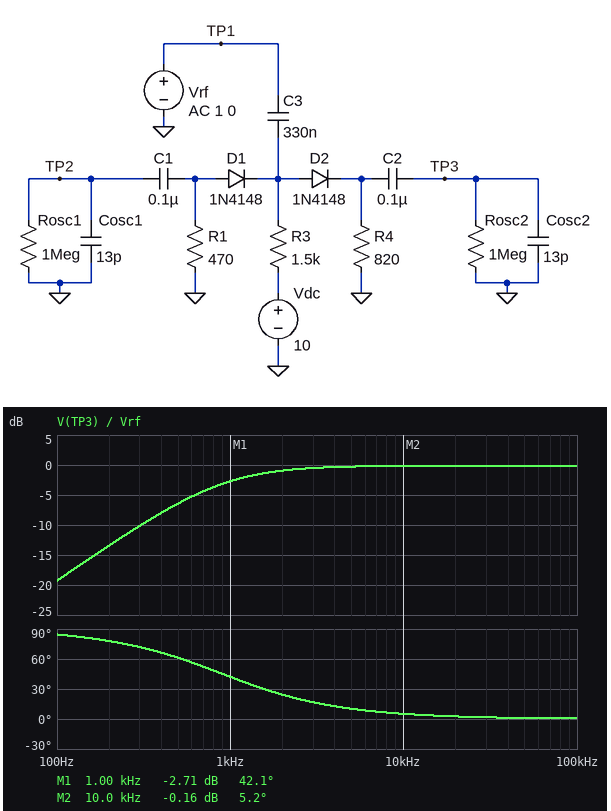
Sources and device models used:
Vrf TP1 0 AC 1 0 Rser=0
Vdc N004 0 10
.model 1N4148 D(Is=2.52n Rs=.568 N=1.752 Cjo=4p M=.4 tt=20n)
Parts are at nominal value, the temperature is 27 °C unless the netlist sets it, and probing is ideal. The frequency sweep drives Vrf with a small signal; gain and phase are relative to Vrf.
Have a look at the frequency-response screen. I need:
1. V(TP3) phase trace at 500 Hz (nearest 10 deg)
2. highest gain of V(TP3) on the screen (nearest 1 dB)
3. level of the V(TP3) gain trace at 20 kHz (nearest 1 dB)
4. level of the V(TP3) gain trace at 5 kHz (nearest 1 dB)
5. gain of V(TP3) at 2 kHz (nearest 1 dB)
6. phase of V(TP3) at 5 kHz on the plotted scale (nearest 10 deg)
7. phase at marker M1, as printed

60 deg
0 dB
0 dB
0 dB
-1 dB
10 deg
42.1 deg
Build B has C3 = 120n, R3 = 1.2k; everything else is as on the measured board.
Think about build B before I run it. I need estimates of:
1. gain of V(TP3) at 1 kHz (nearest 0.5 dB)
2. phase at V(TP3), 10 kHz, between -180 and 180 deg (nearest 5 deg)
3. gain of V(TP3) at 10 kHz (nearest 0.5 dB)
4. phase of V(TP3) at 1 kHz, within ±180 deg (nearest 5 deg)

-9.5 dB
15 deg
-0.5 dB
70 deg
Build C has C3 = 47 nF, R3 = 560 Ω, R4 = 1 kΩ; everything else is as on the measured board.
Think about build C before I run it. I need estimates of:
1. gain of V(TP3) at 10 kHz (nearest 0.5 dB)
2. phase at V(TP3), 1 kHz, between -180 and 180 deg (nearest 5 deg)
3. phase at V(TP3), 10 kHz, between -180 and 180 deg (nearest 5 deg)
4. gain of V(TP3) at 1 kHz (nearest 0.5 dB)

-3.0 dB
85 deg
45 deg
-19.5 dB
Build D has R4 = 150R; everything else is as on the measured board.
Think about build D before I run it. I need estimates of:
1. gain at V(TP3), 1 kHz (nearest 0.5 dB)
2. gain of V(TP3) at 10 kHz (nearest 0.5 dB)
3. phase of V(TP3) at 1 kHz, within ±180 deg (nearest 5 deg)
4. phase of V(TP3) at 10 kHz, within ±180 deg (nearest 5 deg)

-11.5 dB
-1.0 dB
75 deg
20 deg
